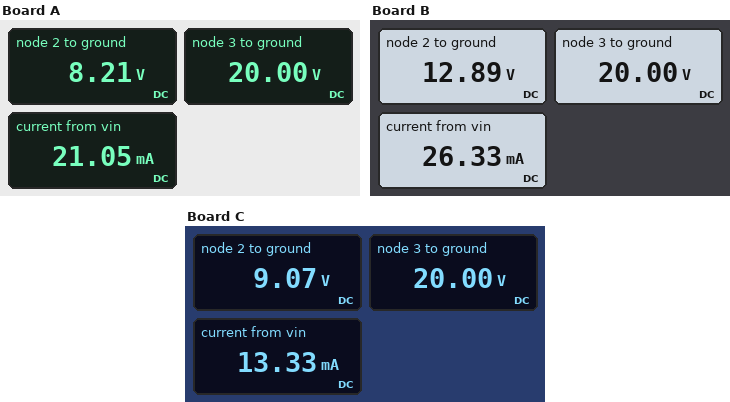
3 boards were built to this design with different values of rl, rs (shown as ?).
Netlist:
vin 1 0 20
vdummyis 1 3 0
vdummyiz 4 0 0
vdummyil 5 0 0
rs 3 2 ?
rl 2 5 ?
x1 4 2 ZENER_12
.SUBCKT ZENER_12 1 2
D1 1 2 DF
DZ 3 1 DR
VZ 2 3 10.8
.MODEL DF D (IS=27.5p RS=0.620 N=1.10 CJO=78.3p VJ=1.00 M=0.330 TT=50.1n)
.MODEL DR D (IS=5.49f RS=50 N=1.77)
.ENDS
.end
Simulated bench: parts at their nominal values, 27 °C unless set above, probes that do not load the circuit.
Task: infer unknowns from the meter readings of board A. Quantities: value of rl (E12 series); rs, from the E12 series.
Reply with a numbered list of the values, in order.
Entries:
1. 390 Ω
2. 560 Ω
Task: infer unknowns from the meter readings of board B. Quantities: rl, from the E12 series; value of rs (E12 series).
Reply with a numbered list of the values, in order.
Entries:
1. 1.2 kΩ
2. 270 Ω
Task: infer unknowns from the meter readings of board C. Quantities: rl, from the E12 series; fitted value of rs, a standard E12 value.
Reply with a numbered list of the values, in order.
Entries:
1. 680 Ω
2. 820 Ω
